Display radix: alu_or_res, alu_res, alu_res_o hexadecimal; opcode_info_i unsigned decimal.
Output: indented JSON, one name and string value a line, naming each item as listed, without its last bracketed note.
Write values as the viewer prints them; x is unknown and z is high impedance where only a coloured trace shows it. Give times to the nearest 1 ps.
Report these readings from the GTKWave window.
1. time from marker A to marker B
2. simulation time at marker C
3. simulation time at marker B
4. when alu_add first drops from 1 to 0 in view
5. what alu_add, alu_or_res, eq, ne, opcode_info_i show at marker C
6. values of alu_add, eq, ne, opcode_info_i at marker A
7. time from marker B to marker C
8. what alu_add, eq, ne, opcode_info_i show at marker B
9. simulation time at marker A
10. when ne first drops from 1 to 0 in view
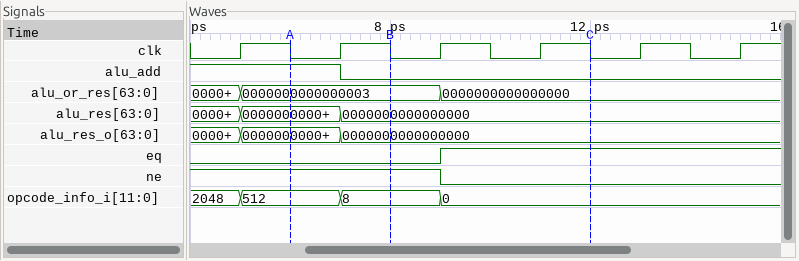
{
  "time from marker A to marker B": "2 ps",
  "simulation time at marker C": "12 ps",
  "simulation time at marker B": "8 ps",
  "when alu_add first drops from 1 to 0 in view": "7 ps",
  "what alu_add, alu_or_res, eq, ne, opcode_info_i show at marker C": "alu_add=0, alu_or_res=0000000000000000, eq=1, ne=0, opcode_info_i=0",
  "values of alu_add, eq, ne, opcode_info_i at marker A": "alu_add=1, eq=0, ne=1, opcode_info_i=512",
  "time from marker B to marker C": "4 ps",
  "what alu_add, eq, ne, opcode_info_i show at marker B": "alu_add=0, eq=0, ne=1, opcode_info_i=8",
  "simulation time at marker A": "6 ps",
  "when ne first drops from 1 to 0 in view": "9 ps"
}
